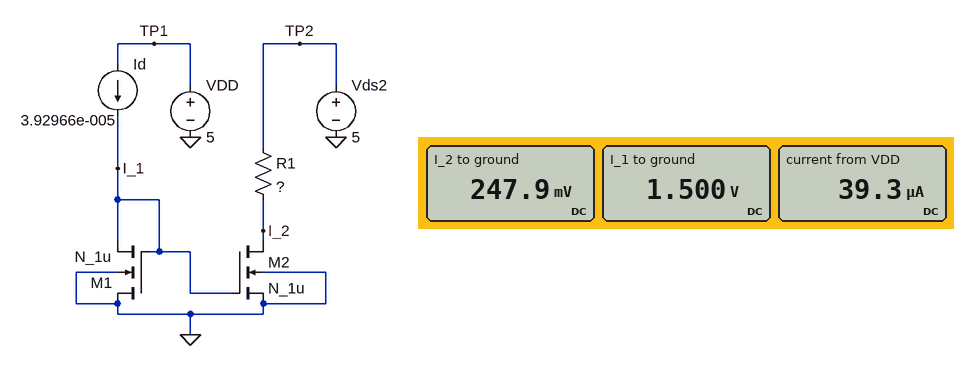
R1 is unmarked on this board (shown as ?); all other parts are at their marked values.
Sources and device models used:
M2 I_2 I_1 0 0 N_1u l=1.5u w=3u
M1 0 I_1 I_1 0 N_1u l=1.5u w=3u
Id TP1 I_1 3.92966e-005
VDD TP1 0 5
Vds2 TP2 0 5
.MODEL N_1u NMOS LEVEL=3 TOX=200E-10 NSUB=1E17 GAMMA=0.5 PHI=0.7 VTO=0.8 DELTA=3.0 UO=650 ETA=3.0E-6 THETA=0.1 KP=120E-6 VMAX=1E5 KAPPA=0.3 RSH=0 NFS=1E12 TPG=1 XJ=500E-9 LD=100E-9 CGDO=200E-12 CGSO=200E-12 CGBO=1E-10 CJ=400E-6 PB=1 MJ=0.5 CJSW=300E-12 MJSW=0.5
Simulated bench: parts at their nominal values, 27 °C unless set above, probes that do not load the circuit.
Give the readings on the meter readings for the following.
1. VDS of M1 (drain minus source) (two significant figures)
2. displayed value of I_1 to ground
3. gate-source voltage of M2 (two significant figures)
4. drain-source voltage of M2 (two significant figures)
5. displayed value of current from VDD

-1.5 V
1.500 V
1.5 V
250 mV
39.3 µA
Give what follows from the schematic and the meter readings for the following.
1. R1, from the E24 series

160 kΩ
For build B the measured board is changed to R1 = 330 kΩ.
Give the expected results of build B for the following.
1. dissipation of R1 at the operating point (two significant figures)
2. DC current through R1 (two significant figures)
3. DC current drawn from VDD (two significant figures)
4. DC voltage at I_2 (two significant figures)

73 µW
15 µA
39 µA
99 mV
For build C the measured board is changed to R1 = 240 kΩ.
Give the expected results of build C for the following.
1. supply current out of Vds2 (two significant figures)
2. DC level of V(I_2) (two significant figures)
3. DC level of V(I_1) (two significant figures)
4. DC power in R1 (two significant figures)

20 µA
140 mV
1.5 V
98 µW
